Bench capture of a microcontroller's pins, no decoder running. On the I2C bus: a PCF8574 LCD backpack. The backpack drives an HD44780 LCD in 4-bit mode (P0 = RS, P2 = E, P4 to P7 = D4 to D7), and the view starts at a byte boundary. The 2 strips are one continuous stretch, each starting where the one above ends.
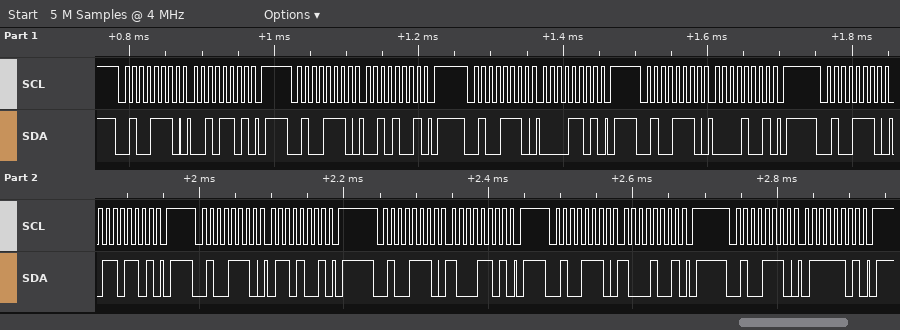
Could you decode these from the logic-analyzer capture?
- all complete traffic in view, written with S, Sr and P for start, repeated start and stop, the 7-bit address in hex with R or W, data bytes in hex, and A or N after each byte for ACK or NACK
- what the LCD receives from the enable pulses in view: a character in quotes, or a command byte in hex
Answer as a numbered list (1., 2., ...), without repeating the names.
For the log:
1. S 27W A 2D A P S 27W A 29 A P S 27W A 0D A P S 27W A 09 A P S 27W A 6D A P S 27W A 69 A P S 27W A 8D A P S 27W A 89 A P S 27W A 7D A P
2. ' ' 'h'
